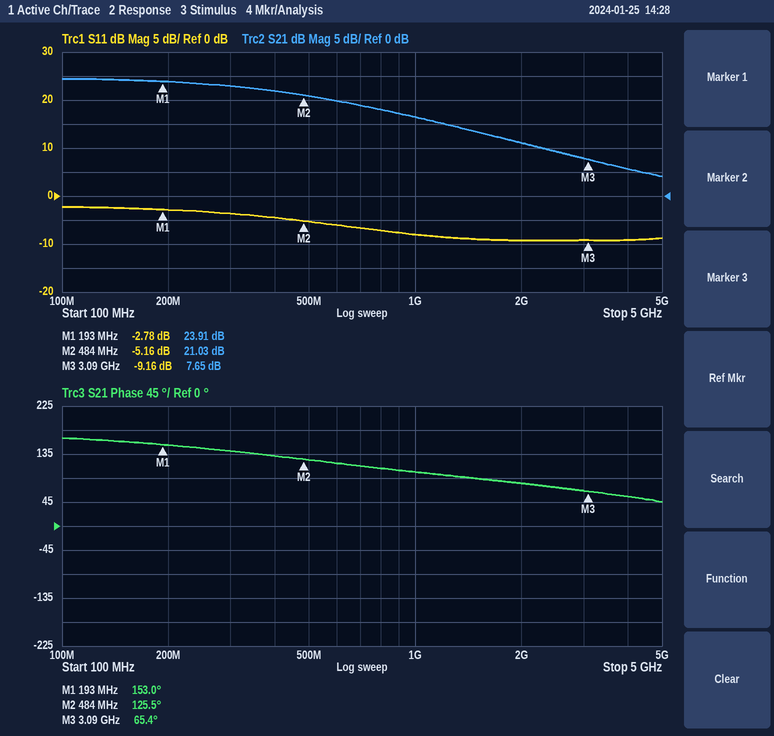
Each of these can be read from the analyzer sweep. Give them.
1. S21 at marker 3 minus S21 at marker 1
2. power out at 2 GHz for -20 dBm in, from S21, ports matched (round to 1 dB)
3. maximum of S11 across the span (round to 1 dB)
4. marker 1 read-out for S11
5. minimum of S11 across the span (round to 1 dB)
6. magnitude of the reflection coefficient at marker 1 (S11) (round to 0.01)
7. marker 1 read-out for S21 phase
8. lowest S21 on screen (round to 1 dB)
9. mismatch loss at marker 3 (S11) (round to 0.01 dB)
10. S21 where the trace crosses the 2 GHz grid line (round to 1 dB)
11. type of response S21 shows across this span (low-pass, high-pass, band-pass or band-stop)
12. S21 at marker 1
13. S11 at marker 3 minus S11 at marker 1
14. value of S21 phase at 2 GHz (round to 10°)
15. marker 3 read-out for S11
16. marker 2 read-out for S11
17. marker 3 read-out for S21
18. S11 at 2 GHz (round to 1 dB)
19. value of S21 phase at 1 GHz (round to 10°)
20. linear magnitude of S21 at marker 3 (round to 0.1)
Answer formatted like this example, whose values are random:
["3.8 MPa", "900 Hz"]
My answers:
["-16.26 dB", "-9 dBm", "-2 dB", "-2.78 dB", "-9 dB", "0.73", "153.0°", "4 dB", "0.56 dB", "11 dB", "low-pass", "23.91 dB", "-6.38 dB", "80°", "-9.16 dB", "-5.16 dB", "7.65 dB", "-9 dB", "100°", "2.4"]
